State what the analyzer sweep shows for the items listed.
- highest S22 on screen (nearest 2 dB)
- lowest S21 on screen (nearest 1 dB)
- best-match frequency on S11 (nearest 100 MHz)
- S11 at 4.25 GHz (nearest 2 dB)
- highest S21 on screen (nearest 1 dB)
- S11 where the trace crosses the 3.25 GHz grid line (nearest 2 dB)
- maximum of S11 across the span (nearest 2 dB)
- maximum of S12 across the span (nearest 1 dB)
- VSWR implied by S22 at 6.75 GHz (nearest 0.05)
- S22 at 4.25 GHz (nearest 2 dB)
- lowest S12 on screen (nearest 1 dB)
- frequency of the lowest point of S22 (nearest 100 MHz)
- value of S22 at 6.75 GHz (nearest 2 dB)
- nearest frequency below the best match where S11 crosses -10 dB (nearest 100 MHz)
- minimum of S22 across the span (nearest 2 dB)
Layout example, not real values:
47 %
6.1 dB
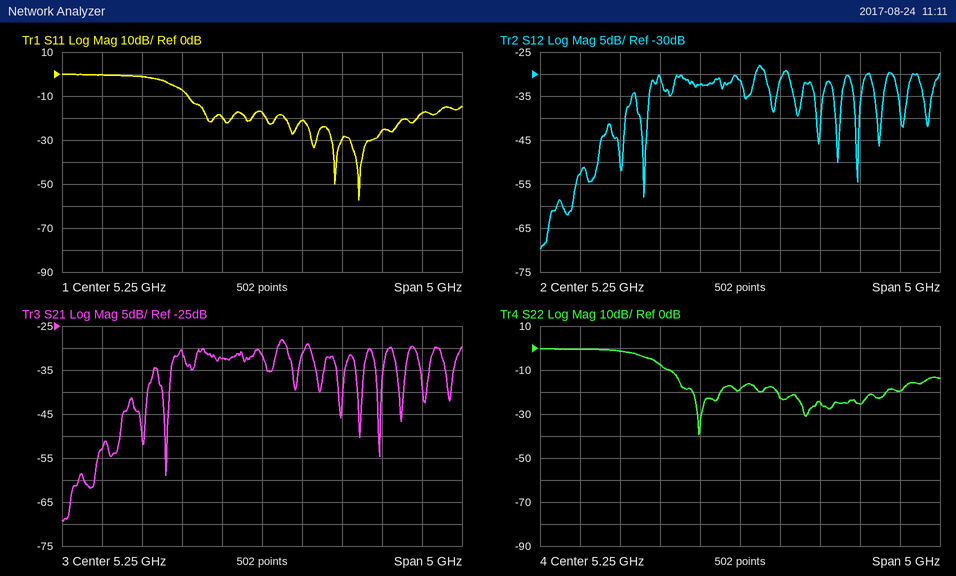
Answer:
0 dB
-69 dB
6.5 GHz
-8 dB
-28 dB
0 dB
0 dB
-28 dB
1.10
-8 dB
-70 dB
4.7 GHz
-26 dB
4.3 GHz
-40 dB
